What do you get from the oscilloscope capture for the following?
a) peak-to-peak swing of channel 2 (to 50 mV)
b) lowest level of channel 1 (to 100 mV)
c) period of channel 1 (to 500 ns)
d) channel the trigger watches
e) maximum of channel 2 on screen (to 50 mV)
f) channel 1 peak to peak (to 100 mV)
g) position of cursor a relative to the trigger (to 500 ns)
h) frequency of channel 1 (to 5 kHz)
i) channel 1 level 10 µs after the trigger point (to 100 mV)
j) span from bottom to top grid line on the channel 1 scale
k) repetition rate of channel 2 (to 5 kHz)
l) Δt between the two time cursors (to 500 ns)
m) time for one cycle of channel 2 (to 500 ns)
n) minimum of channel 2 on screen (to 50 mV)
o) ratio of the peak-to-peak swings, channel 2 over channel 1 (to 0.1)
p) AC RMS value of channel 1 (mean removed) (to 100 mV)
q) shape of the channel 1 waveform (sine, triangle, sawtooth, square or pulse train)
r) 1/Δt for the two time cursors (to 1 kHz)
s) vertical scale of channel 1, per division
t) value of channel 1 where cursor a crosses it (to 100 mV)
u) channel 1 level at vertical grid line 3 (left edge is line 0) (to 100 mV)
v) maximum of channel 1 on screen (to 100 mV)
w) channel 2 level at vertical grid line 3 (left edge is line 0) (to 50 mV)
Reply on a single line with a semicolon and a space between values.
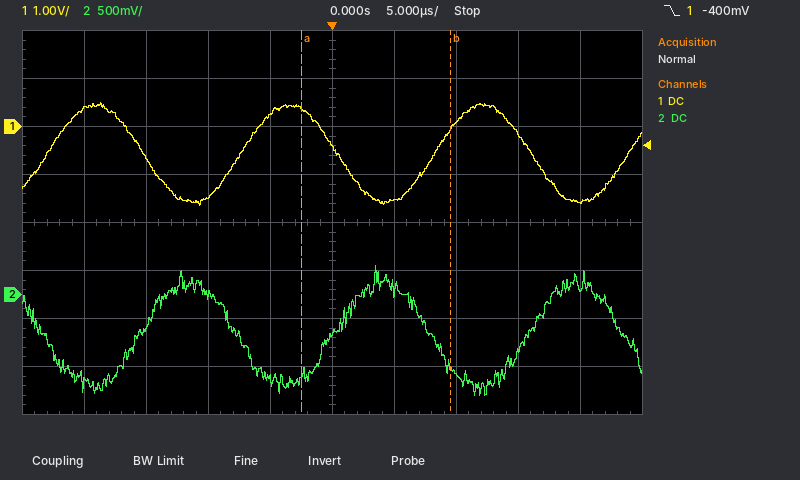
1.35 V; -1.6 V; 15.5 µs; channel 1; 300 mV; 2.1 V; -2.5 µs; 65 kHz; 100 mV; 8 V; 65 kHz; 12.0 µs; 15.5 µs; -1.05 V; 0.6; 700 mV; sine; 83 kHz; 1 V; 400 mV; -1.5 V; 500 mV; 0 mV
